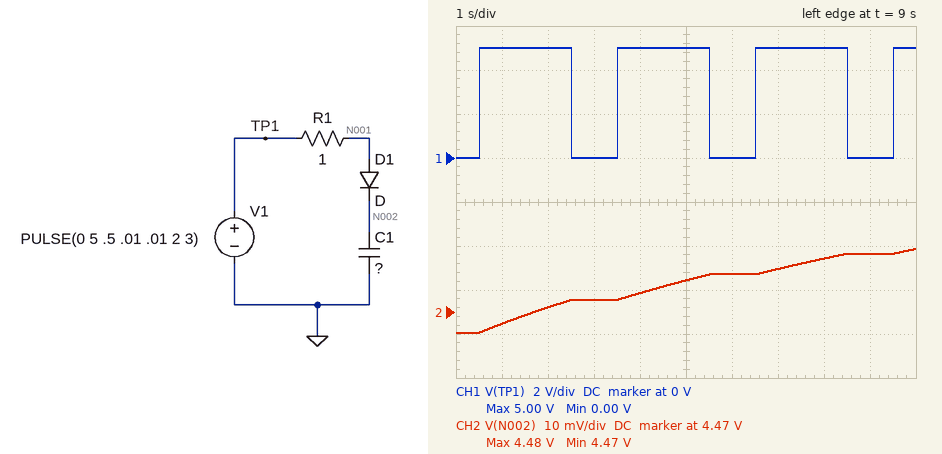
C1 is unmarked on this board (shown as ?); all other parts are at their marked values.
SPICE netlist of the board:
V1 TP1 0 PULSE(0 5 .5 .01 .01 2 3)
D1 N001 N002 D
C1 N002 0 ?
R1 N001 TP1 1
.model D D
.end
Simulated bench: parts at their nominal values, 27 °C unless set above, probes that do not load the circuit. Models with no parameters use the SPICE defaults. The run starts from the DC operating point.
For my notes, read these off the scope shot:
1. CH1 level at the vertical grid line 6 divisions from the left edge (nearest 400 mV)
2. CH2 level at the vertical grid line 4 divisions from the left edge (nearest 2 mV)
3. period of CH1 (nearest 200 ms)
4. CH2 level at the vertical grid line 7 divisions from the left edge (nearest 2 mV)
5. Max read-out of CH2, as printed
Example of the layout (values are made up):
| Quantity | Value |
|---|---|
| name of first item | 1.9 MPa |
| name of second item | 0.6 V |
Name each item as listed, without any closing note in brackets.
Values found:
| Quantity | Value |
|---|---|
| CH1 level at the vertical grid line 6 divisions from the left edge | 0 V |
| CH2 level at the vertical grid line 4 divisions from the left edge | 4.474 V |
| period of CH1 | 3.0 s |
| CH2 level at the vertical grid line 7 divisions from the left edge | 4.480 V |
| Max read-out of CH2, as printed | 4.48 V |
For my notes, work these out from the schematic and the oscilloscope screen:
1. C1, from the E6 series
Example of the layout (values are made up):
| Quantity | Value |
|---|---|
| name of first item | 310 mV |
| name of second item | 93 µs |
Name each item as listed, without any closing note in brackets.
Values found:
| Quantity | Value |
|---|---|
| C1, from the E6 series | 2.2 mF |
